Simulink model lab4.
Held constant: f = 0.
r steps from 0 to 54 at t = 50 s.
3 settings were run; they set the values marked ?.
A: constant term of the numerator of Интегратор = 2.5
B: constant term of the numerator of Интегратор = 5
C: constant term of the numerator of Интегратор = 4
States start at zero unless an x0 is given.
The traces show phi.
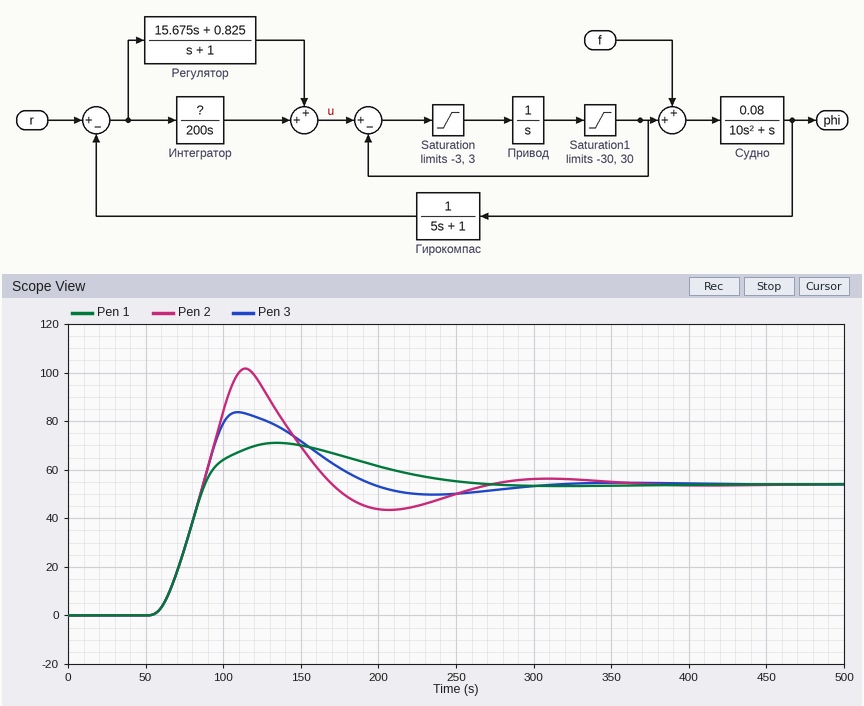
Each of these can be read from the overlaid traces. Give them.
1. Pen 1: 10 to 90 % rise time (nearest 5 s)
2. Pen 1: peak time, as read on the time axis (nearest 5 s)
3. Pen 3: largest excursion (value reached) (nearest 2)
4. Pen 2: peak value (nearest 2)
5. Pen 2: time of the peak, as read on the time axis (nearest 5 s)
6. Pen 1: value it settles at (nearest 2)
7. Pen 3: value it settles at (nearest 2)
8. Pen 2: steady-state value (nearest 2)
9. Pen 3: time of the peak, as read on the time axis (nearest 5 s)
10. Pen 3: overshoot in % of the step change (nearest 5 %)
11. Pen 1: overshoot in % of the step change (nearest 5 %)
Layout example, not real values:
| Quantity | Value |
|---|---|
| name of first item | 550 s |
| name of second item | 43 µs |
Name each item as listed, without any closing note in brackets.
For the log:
| Quantity | Value |
|---|---|
| Pen 1: 10 to 90 % rise time | 25 s |
| Pen 1: peak time, as read on the time axis | 135 s |
| Pen 3: largest excursion (value reached) | 84 |
| Pen 2: peak value | 102 |
| Pen 2: time of the peak, as read on the time axis | 115 s |
| Pen 1: value it settles at | 54 |
| Pen 3: value it settles at | 54 |
| Pen 2: steady-state value | 54 |
| Pen 3: time of the peak, as read on the time axis | 110 s |
| Pen 3: overshoot in % of the step change | 55 % |
| Pen 1: overshoot in % of the step change | 30 % |
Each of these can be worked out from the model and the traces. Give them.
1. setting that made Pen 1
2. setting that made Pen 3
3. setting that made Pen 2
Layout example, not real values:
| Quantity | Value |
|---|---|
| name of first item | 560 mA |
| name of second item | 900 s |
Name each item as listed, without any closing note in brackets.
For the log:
| Quantity | Value |
|---|---|
| setting that made Pen 1 | A |
| setting that made Pen 3 | C |
| setting that made Pen 2 | B |
